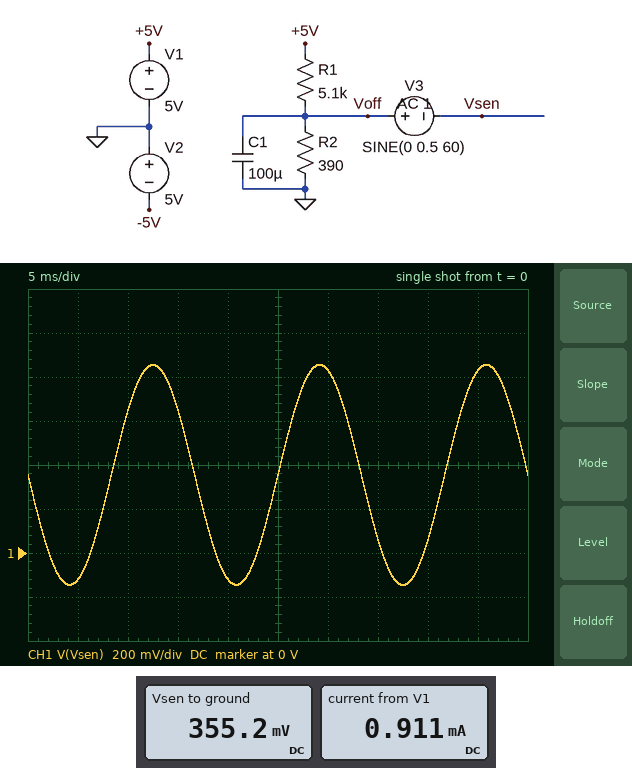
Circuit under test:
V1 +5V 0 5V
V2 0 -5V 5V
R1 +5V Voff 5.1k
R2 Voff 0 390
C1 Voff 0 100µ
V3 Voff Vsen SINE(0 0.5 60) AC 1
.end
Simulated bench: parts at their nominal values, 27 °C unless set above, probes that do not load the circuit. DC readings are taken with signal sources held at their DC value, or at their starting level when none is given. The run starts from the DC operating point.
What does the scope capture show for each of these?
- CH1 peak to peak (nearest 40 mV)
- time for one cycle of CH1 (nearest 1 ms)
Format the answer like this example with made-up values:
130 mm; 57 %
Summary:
1.00 V; 17 ms
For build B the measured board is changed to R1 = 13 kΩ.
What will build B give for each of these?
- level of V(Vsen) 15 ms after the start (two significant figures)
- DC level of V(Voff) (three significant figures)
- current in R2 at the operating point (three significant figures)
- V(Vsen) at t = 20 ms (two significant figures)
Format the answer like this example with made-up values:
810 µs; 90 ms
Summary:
440 mV; 146 mV; 373 µA; -330 mV
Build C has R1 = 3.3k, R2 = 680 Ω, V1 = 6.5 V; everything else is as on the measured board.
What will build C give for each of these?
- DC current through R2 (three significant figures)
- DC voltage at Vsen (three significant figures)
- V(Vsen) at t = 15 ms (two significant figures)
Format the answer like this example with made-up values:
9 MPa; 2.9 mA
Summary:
1.63 mA; 1.11 V; 1.4 V
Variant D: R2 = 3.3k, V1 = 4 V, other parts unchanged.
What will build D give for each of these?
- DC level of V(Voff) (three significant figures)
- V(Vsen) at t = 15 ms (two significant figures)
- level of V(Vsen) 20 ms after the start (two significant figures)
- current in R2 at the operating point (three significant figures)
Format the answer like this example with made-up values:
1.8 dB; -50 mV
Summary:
1.57 V; 1.9 V; 1.1 V; 476 µA
